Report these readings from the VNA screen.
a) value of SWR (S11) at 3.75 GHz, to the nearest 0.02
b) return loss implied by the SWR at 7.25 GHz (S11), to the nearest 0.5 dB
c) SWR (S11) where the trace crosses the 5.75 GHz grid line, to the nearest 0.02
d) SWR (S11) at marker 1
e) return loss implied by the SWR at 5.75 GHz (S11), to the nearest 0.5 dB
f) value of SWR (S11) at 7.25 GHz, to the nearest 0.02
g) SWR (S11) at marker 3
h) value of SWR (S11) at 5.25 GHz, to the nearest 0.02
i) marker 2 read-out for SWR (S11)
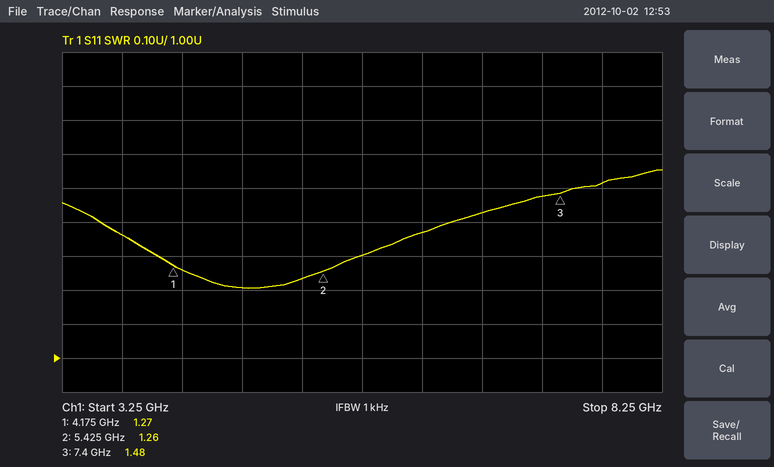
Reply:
1.36
14.5 dB
1.30
1.27
17.5 dB
1.48
1.48
1.24
1.26
